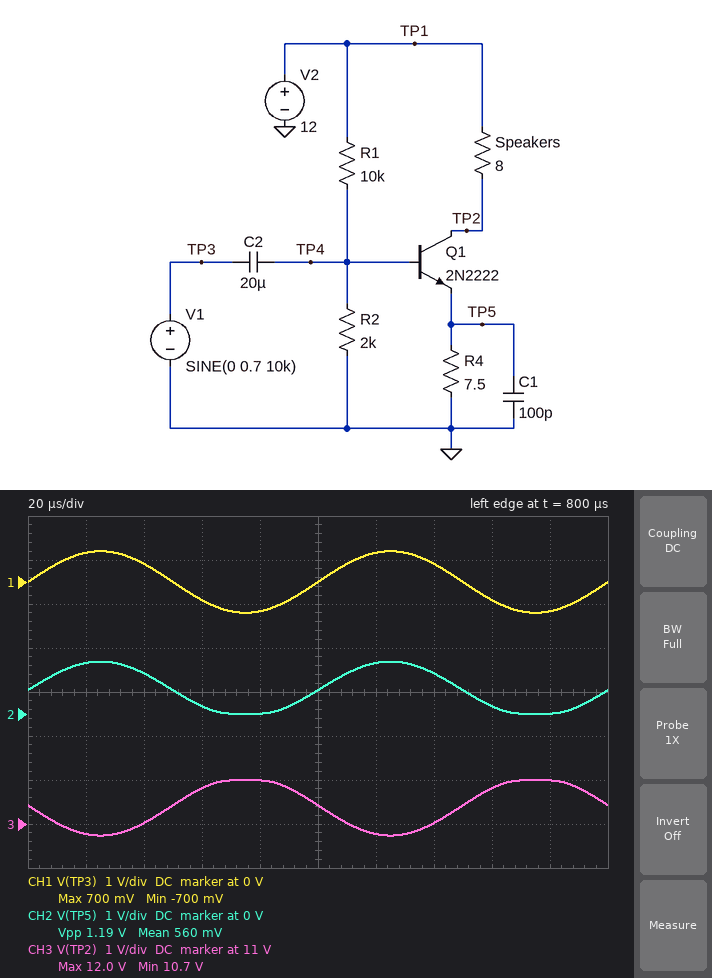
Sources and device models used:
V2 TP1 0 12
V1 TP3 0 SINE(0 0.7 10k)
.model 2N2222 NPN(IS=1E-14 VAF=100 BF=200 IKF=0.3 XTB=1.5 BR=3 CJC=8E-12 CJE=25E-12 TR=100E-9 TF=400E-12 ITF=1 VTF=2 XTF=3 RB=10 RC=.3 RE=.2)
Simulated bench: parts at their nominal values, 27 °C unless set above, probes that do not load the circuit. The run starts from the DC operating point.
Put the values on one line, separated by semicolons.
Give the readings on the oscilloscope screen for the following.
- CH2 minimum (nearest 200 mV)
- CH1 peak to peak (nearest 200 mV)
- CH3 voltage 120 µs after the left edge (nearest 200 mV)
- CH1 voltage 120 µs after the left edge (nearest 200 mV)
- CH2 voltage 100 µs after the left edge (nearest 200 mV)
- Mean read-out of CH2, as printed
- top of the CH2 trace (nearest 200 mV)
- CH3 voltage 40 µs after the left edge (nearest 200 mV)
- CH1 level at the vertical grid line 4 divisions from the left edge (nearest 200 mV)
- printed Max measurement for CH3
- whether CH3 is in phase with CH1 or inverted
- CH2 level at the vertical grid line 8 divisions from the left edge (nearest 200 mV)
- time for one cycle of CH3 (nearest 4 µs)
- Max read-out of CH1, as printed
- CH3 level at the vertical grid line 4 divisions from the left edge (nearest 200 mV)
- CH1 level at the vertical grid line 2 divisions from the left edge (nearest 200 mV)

0 V; 1.4 V; 10.8 V; 600 mV; 600 mV; 560 mV; 1.2 V; 11.0 V; -600 mV; 12.0 V; inverted; 200 mV; 100 µs; 700 mV; 12.0 V; 400 mV
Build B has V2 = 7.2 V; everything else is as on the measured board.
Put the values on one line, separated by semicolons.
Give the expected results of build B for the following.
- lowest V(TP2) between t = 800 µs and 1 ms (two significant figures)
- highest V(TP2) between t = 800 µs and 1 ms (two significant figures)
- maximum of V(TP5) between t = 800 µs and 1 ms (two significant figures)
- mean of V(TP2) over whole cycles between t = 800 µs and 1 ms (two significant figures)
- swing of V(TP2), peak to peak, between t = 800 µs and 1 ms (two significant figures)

6.3 V; 7.2 V; 840 mV; 6.9 V; 890 mV
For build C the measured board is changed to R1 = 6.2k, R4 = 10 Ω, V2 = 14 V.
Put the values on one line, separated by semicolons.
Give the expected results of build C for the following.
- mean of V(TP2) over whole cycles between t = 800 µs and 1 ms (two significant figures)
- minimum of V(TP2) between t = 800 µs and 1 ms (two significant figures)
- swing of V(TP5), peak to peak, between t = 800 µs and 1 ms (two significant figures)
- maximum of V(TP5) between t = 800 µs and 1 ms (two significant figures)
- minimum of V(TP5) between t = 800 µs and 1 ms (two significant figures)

13 V; 12 V; 1.3 V; 2.0 V; 670 mV
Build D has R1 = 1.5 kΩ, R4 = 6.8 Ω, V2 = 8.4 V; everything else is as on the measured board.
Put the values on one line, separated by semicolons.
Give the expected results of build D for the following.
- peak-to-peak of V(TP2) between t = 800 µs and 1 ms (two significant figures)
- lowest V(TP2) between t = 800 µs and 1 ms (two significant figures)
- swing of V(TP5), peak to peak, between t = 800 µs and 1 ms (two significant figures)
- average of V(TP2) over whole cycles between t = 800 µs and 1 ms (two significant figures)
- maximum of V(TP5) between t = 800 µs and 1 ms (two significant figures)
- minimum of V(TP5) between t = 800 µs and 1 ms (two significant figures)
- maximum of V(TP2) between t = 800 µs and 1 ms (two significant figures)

1.5 V; 5.5 V; 1.3 V; 6.3 V; 2.5 V; 1.2 V; 7.0 V
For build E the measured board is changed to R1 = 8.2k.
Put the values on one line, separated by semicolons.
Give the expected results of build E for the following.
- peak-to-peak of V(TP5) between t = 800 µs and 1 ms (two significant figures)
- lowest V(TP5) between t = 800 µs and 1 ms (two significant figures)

1.3 V; 74 mV
